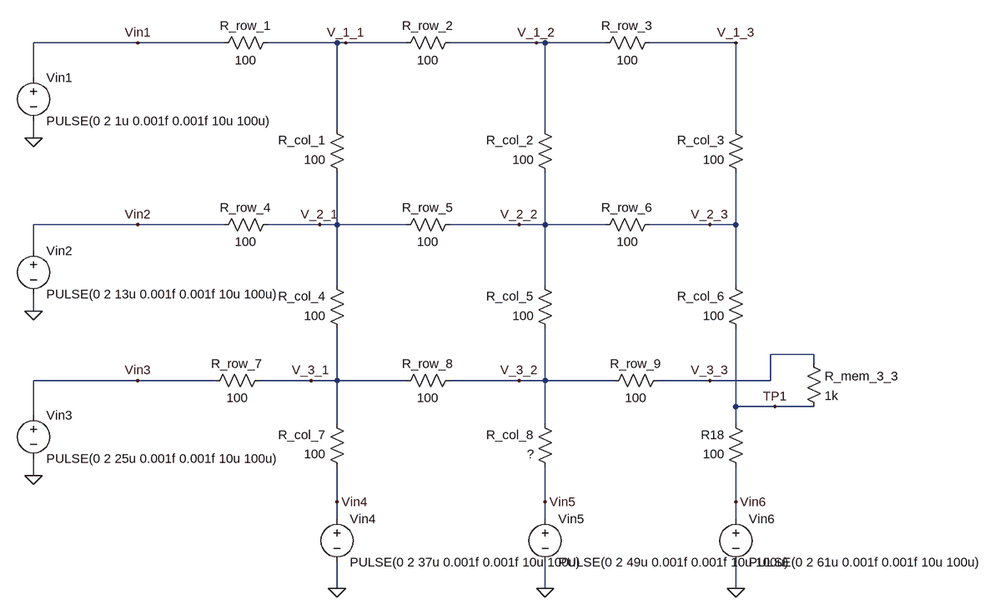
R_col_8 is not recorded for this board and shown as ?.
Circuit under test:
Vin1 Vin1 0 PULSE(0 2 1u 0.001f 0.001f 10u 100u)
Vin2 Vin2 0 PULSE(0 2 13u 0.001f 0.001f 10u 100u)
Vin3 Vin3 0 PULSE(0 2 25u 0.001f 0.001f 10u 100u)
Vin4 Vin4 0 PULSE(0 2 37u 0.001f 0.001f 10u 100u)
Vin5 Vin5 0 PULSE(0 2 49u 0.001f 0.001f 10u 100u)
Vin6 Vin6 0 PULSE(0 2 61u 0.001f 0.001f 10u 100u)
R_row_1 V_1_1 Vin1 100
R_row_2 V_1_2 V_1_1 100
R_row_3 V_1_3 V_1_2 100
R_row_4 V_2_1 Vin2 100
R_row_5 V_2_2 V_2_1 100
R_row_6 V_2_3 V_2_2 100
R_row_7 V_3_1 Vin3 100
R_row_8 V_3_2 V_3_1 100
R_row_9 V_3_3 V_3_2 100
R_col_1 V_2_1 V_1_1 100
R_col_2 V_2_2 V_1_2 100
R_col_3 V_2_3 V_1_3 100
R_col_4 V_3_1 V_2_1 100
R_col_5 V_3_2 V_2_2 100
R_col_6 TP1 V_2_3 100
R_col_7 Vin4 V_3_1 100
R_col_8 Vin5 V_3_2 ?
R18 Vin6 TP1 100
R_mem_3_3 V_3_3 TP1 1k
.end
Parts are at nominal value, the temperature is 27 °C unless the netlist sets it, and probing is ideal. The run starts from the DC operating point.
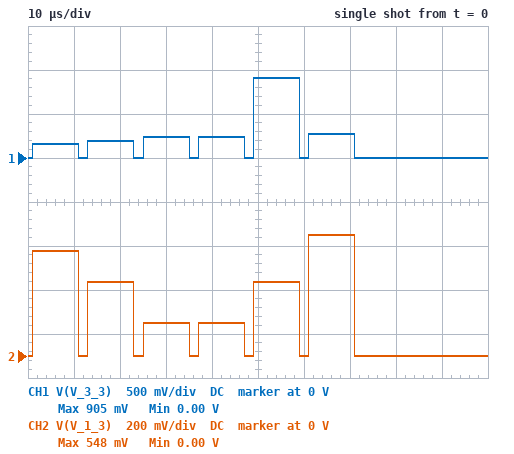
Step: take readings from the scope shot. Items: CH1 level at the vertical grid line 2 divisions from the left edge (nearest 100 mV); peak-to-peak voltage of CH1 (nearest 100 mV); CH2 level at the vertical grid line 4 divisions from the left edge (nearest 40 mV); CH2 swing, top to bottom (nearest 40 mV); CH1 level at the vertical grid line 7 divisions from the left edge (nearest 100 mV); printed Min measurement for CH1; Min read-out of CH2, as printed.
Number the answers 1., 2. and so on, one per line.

1. 200 mV
2. 900 mV
3. 160 mV
4. 560 mV
5. 300 mV
6. 0.00 V
7. 0.00 V
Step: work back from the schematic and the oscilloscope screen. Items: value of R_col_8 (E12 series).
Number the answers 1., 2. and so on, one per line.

1. 82 Ω
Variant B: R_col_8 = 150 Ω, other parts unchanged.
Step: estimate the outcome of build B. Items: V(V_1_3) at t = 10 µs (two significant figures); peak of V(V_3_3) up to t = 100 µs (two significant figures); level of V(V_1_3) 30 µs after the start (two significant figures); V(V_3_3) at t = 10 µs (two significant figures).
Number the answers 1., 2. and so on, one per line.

1. 490 mV
2. 640 mV
3. 180 mV
4. 200 mV
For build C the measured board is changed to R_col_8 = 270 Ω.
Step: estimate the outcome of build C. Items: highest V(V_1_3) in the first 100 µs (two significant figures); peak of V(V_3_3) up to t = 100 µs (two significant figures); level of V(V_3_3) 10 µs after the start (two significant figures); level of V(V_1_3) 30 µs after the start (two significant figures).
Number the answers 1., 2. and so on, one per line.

1. 580 mV
2. 420 mV
3. 230 mV
4. 200 mV
